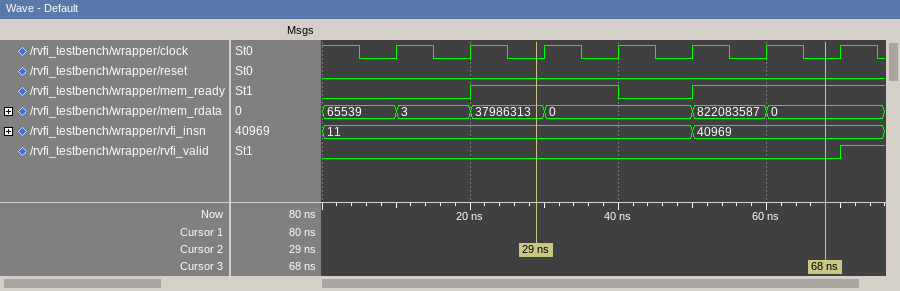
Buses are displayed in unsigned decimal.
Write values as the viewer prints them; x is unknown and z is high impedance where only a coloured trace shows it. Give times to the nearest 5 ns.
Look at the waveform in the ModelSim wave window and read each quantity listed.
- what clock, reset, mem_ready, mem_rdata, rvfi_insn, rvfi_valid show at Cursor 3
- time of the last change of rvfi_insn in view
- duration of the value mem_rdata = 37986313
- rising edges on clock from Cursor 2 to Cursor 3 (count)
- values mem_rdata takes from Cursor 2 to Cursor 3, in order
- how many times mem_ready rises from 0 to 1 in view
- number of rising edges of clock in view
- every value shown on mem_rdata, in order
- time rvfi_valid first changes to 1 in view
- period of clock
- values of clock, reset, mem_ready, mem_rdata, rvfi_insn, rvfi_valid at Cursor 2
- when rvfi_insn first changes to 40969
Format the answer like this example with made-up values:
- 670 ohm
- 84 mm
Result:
- clock=0, reset=0, mem_ready=1, mem_rdata=0, rvfi_insn=40969, rvfi_valid=0
- 50 ns
- 10 ns
- 4
- 37986313, 0, 822083587, 0
- 2
- 7
- 65539, 3, 37986313, 0, 822083587, 0
- 70 ns
- 10 ns
- clock=0, reset=0, mem_ready=1, mem_rdata=37986313, rvfi_insn=11, rvfi_valid=0
- 50 ns
